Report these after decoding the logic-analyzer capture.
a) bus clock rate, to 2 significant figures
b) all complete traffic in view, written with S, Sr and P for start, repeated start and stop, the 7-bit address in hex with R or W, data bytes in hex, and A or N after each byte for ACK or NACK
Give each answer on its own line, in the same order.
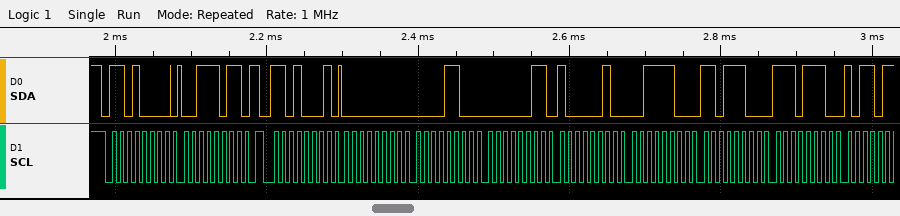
100 kHz
S 68W A 3B A Sr 68R A 00 A 0C A 03 A 82 A 3C A DC A EE A
